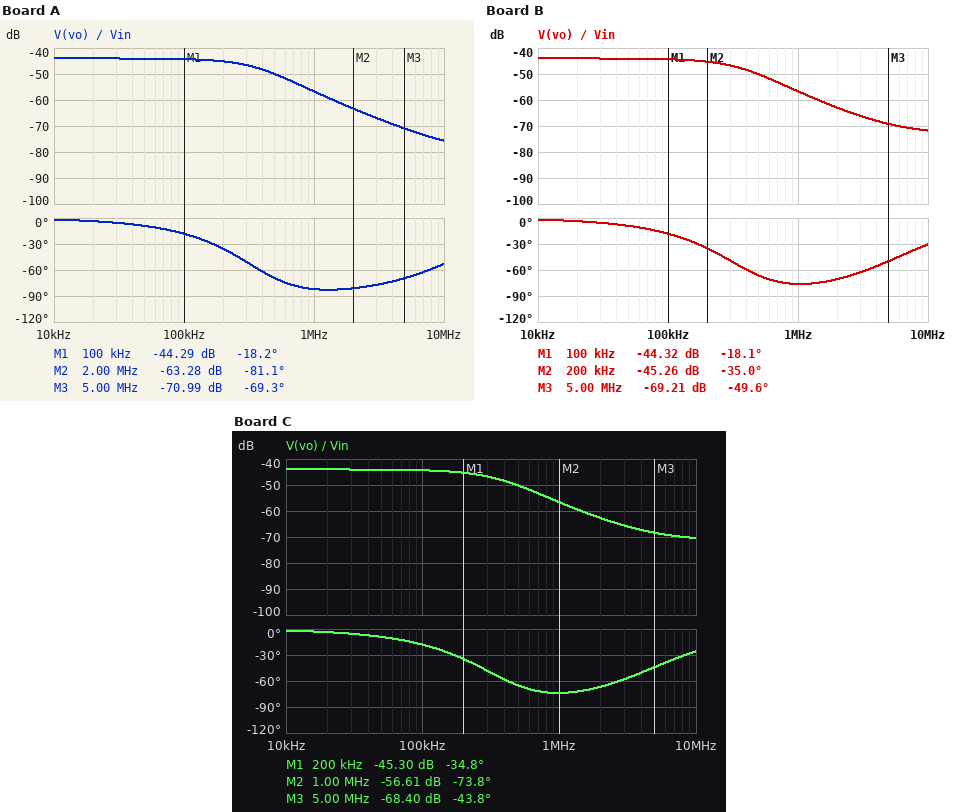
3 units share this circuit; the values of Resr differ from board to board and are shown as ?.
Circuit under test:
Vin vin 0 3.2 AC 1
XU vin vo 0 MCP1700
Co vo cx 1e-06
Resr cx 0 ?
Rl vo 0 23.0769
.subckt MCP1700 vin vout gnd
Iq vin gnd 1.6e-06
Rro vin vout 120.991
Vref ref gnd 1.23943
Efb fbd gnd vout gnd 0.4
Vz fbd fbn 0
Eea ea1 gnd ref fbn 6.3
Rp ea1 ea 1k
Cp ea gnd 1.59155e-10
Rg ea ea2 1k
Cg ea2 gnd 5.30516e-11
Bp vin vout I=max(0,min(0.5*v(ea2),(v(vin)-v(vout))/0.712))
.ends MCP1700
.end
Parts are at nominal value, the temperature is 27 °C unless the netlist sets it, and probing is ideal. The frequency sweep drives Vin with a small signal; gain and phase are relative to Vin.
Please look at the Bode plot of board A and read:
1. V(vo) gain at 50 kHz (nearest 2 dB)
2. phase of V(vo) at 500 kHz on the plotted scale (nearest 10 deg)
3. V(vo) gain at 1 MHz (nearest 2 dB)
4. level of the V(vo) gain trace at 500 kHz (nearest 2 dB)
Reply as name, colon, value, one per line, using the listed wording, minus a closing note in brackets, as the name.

V(vo) gain at 50 kHz: -44 dB
phase of V(vo) at 500 kHz on the plotted scale: -70 deg
V(vo) gain at 1 MHz: -56 dB
level of the V(vo) gain trace at 500 kHz: -50 dB
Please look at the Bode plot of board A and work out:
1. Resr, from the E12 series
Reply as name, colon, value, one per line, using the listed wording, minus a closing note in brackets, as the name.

Resr, from the E12 series: 0.012 Ω
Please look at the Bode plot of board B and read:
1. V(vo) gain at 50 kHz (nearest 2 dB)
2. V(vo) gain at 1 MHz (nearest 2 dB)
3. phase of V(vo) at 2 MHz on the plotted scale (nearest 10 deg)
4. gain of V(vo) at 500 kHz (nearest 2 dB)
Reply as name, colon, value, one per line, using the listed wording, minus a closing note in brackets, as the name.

V(vo) gain at 50 kHz: -44 dB
V(vo) gain at 1 MHz: -56 dB
phase of V(vo) at 2 MHz on the plotted scale: -70 deg
gain of V(vo) at 500 kHz: -50 dB
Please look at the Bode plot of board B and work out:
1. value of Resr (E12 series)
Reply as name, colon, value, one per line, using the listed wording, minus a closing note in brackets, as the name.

value of Resr: 0.027 Ω
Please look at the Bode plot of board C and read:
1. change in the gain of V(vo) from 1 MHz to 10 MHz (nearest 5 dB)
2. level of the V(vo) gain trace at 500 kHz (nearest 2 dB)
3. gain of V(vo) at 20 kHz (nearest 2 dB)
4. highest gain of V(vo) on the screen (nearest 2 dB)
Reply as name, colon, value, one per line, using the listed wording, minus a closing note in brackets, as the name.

change in the gain of V(vo) from 1 MHz to 10 MHz: -15 dB
level of the V(vo) gain trace at 500 kHz: -50 dB
gain of V(vo) at 20 kHz: -44 dB
highest gain of V(vo) on the screen: -44 dB
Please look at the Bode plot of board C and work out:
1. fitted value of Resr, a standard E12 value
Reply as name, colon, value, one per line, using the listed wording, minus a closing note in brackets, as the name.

fitted value of Resr, a standard E12 value: 0.033 Ω
